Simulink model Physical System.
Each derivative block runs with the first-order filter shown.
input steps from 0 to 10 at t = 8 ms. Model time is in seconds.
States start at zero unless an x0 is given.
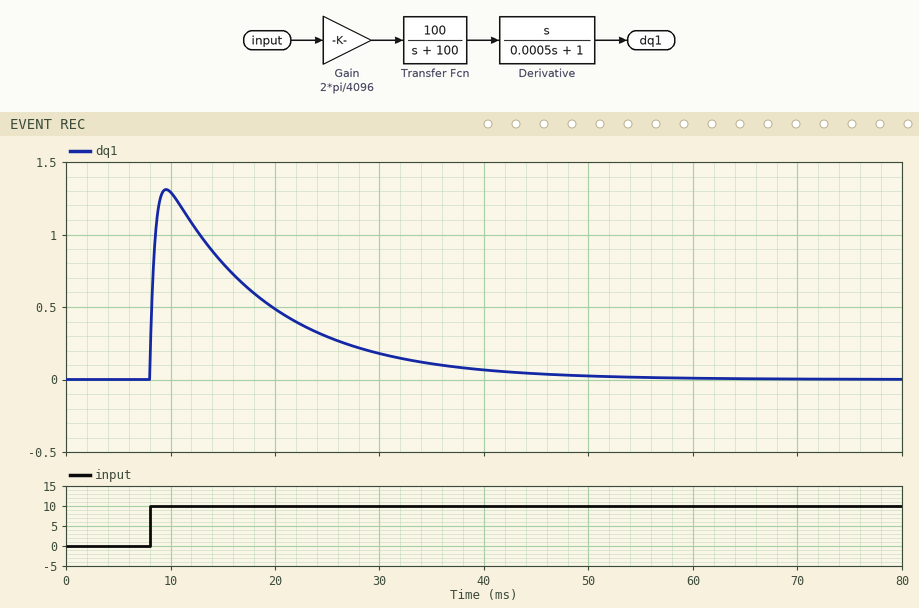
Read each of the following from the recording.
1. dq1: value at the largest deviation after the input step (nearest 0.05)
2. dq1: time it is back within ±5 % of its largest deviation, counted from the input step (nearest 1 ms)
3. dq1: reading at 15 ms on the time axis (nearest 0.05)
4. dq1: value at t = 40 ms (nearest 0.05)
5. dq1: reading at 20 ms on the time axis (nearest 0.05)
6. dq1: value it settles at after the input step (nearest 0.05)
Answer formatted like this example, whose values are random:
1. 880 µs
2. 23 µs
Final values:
1. 1.30
2. 32 ms
3. 0.80
4. 0.05
5. 0.50
6. 0.00
